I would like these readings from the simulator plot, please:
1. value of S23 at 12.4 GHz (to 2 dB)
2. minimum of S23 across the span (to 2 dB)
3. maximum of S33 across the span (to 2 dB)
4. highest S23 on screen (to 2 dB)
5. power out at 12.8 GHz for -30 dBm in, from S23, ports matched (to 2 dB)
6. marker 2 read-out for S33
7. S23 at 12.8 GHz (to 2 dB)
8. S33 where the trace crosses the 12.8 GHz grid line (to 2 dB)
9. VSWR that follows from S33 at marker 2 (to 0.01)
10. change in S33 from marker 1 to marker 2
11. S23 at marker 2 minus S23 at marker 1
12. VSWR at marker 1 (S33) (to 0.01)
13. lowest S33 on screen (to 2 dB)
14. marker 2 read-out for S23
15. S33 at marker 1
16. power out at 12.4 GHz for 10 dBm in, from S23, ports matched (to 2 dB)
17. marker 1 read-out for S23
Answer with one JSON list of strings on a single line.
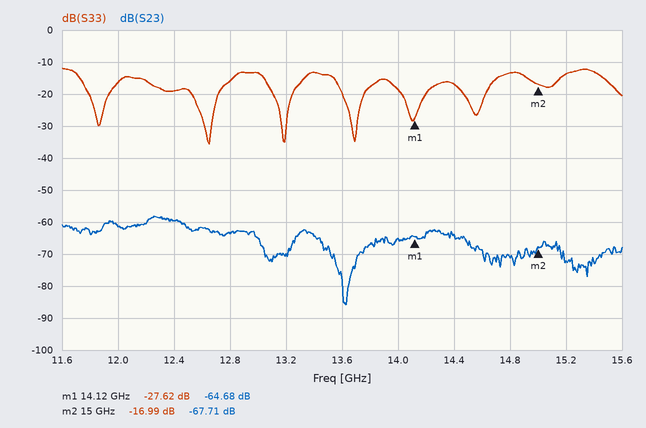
["-60 dB", "-86 dB", "-12 dB", "-58 dB", "-94 dBm", "-16.99 dB", "-64 dB", "-16 dB", "1.33", "10.63 dB", "-3.03 dB", "1.09", "-36 dB", "-67.71 dB", "-27.62 dB", "-50 dBm", "-64.68 dB"]
